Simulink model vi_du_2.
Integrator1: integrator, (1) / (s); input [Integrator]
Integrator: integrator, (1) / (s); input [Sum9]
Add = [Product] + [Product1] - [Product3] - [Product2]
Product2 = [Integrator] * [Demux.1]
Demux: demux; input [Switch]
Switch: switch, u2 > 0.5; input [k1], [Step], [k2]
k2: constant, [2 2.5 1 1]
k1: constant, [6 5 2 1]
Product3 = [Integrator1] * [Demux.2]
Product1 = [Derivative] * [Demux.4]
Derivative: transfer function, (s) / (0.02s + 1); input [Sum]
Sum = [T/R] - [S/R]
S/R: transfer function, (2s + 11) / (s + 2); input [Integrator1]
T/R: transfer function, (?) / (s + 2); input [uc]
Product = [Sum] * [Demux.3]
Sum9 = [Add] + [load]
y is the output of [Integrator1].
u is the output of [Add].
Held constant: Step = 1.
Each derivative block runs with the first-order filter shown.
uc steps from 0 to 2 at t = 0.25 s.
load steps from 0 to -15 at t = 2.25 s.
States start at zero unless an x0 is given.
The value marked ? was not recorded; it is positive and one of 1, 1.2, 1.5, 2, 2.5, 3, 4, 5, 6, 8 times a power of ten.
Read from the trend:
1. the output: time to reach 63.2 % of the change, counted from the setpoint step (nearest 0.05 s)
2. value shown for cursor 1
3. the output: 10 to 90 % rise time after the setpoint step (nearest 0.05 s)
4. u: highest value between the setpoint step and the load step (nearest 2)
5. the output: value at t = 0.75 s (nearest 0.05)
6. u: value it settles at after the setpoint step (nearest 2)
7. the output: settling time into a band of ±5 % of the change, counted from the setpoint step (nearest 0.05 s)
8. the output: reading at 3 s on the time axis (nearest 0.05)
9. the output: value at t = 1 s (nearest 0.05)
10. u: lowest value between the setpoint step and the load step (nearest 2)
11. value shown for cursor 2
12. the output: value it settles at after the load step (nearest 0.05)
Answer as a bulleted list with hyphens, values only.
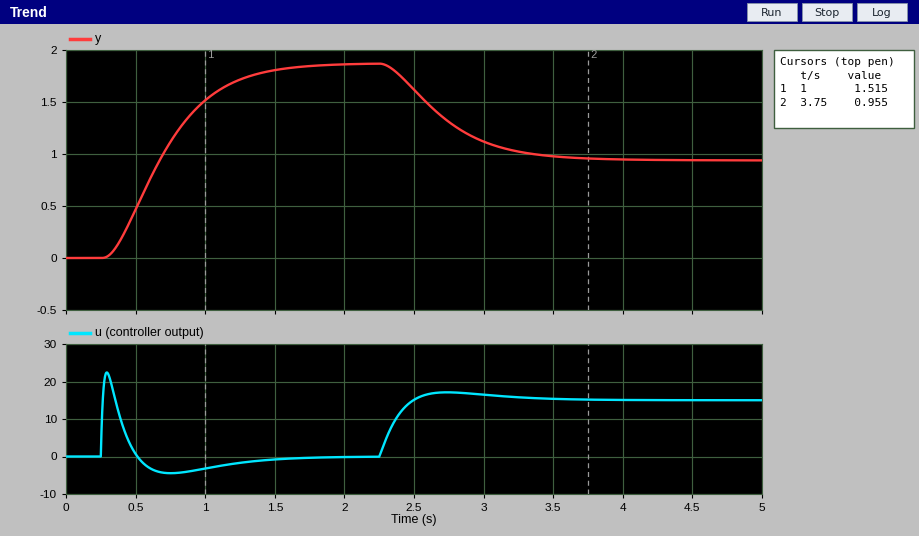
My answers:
- 0.55 s
- 1.515
- 0.80 s
- 22
- 1.10
- 0
- 1.15 s
- 1.10
- 1.50
- -4
- 0.955
- 0.95
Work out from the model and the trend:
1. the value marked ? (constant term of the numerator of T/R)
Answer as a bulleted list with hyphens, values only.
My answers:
- 15
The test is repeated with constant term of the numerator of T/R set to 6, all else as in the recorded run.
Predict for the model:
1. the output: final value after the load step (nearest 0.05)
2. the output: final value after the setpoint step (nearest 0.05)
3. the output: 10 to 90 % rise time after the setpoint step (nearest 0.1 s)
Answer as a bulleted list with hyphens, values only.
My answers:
- -0.20
- 0.75
- 0.8 s
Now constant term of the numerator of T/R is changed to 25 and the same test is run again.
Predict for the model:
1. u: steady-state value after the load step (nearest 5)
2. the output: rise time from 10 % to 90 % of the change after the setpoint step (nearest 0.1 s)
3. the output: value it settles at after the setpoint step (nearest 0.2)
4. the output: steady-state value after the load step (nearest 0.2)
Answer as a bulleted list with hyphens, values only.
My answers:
- 15
- 0.8 s
- 3.2
- 2.2
